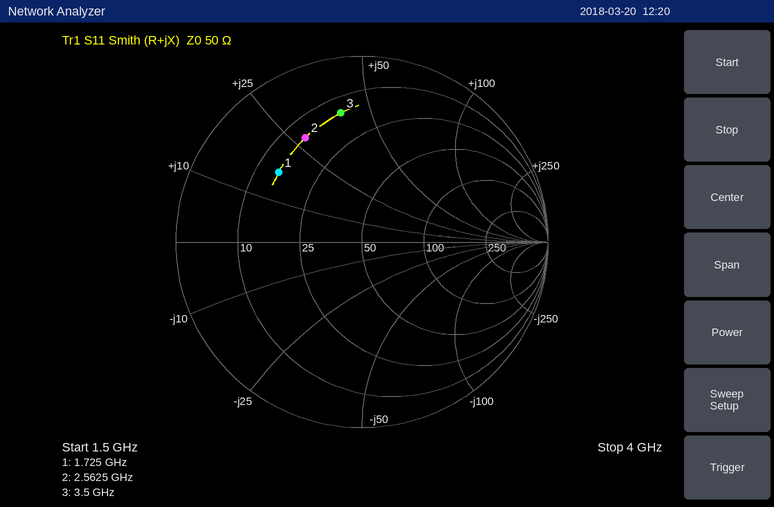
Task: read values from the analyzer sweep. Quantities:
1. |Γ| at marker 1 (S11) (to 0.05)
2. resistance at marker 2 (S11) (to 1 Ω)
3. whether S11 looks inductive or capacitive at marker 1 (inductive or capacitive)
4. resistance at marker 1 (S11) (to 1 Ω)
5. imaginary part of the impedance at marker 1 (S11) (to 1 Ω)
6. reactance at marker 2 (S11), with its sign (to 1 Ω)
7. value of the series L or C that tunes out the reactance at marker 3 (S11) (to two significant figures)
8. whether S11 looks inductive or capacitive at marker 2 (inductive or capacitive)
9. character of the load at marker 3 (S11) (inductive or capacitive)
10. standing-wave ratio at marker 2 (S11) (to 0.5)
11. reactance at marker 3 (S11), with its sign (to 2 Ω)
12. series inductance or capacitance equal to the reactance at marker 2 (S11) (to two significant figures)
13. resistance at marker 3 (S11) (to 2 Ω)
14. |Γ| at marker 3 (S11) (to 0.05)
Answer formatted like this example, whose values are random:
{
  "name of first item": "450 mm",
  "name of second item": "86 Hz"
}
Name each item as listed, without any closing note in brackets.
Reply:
{
  "|Γ| at marker 1 (S11)": "0.60",
  "resistance at marker 2 (S11)": "15 Ω",
  "whether S11 looks inductive or capacitive at marker 1": "inductive",
  "resistance at marker 1 (S11)": "15 Ω",
  "imaginary part of the impedance at marker 1 (S11)": "+17 Ω",
  "reactance at marker 2 (S11), with its sign": "+28 Ω",
  "value of the series L or C that tunes out the reactance at marker 3 (S11)": "1.1 pF",
  "whether S11 looks inductive or capacitive at marker 2": "inductive",
  "character of the load at marker 3 (S11)": "inductive",
  "standing-wave ratio at marker 2 (S11)": "4.5",
  "reactance at marker 3 (S11), with its sign": "+40 Ω",
  "series inductance or capacitance equal to the reactance at marker 2 (S11)": "1.7 nH",
  "resistance at marker 3 (S11)": "14 Ω",
  "|Γ| at marker 3 (S11)": "0.70"
}
